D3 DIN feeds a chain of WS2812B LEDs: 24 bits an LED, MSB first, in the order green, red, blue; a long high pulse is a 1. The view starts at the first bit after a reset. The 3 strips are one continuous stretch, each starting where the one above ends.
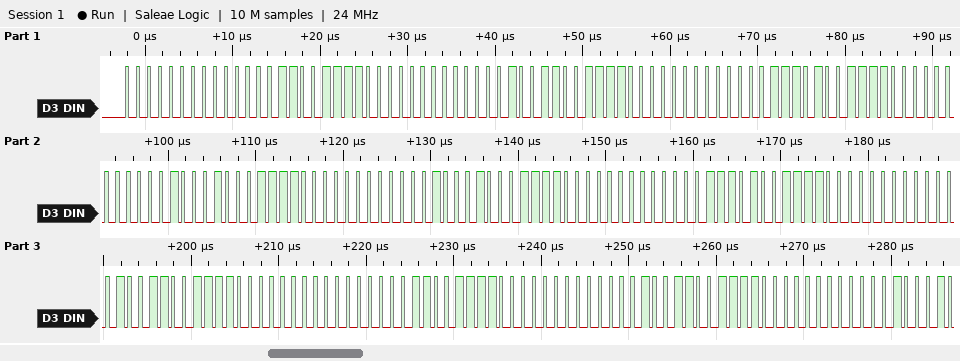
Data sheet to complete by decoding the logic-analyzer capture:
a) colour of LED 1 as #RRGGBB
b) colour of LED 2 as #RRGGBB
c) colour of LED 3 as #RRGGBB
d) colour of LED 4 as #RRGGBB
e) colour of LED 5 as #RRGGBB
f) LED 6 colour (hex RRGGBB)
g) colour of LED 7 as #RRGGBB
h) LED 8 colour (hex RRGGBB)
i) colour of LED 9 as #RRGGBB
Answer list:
#03003C
#13003C
#1D003C
#22003C
#22003C
#1D003C
#13003C
#03003C
#13003C
